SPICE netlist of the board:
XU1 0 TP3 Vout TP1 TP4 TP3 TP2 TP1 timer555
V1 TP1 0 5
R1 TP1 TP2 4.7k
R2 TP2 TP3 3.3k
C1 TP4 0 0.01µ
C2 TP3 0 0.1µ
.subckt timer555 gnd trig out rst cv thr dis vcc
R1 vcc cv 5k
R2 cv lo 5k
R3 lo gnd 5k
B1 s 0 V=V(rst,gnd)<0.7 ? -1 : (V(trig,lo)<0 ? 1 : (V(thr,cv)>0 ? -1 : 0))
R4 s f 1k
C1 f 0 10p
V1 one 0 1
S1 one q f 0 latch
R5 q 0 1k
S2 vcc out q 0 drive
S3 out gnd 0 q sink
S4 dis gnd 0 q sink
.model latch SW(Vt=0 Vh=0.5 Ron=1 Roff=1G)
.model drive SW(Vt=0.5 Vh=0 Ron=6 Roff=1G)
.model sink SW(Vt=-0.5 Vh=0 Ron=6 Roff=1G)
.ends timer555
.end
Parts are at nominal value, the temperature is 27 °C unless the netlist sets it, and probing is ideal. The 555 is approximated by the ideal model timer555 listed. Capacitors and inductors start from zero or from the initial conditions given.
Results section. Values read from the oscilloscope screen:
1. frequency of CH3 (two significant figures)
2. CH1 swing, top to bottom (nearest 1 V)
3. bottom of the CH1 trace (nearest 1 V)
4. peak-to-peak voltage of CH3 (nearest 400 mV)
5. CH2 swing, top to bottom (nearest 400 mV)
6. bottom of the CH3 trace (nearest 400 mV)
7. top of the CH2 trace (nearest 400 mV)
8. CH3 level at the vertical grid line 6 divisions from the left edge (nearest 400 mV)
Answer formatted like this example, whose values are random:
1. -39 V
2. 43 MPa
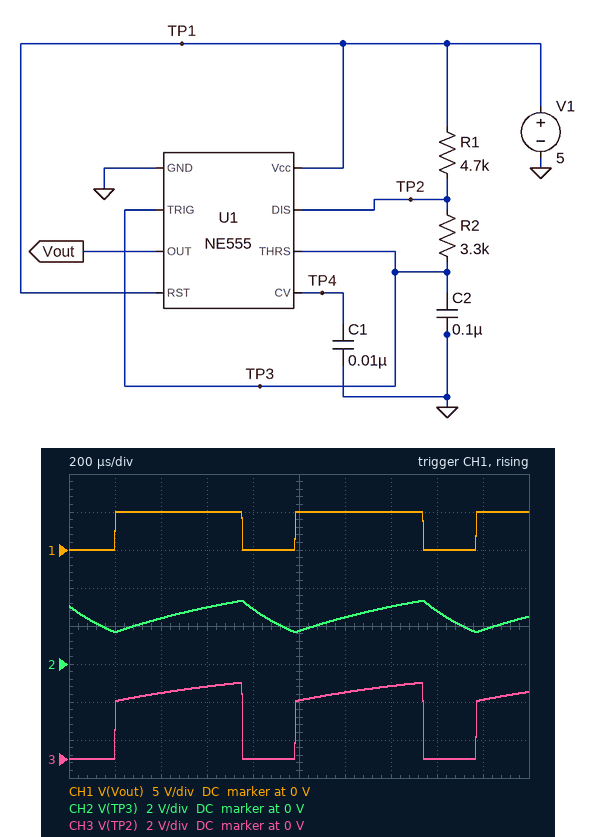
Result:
1. 1.3 kHz
2. 5 V
3. 0 V
4. 4.0 V
5. 1.6 V
6. 0 V
7. 3.2 V
8. 3.6 V
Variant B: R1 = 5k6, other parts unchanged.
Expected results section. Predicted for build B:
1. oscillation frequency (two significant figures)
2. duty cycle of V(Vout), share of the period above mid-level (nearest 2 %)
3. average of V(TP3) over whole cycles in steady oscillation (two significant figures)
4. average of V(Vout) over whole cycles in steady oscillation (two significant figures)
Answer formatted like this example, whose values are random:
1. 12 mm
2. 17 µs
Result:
1. 1.2 kHz
2. 72 %
3. 2.5 V
4. 3.6 V
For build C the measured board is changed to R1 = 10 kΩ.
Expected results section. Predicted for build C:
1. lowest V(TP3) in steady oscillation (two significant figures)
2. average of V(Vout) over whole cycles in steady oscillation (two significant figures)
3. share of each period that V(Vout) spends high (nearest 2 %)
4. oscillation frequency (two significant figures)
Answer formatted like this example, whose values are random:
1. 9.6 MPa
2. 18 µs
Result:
1. 1.7 V
2. 4.0 V
3. 80 %
4. 870 Hz
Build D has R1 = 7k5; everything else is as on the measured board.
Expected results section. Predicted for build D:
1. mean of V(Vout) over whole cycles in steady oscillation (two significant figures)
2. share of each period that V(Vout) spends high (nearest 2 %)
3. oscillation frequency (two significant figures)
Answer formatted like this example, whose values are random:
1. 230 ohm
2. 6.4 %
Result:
1. 3.8 V
2. 76 %
3. 1.0 kHz
